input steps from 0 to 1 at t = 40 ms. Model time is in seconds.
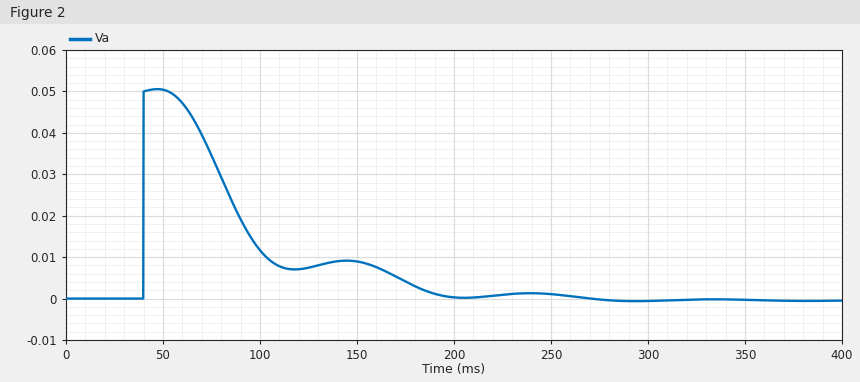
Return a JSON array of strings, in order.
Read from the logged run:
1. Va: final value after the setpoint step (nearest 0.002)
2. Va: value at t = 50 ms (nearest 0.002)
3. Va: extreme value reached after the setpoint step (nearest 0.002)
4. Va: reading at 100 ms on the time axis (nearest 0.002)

["0.000", "0.050", "0.050", "0.012"]
